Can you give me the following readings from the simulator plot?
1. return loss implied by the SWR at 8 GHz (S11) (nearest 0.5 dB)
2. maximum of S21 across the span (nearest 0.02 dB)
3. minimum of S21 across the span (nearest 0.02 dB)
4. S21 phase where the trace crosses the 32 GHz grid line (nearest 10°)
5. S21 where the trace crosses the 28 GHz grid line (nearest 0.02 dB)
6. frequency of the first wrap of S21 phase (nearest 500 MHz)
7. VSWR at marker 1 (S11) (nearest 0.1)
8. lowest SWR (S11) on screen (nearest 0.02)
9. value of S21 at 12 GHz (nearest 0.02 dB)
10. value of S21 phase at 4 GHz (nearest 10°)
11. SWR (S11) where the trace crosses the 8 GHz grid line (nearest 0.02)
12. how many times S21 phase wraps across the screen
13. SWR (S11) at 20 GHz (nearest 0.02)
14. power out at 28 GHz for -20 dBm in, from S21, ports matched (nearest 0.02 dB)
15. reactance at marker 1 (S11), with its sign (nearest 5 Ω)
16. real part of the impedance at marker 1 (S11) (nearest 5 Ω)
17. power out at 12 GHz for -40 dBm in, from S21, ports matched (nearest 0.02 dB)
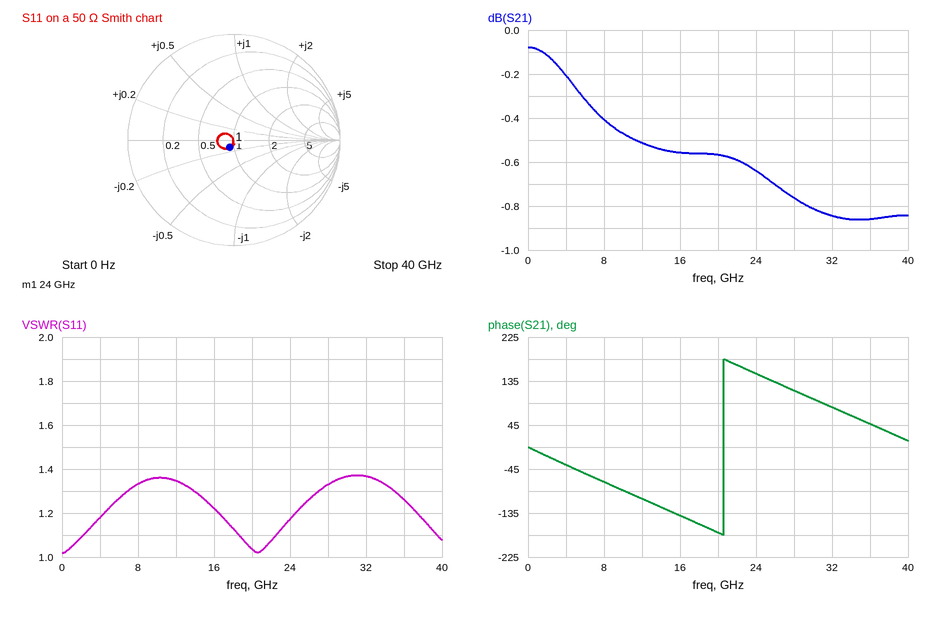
17.0 dB
-0.08 dB
-0.86 dB
80°
-0.76 dB
20.5 GHz
1.2
1.02
-0.52 dB
-40°
1.34
1
1.04
-20.76 dBm
-5 Ω
45 Ω
-40.52 dBm
